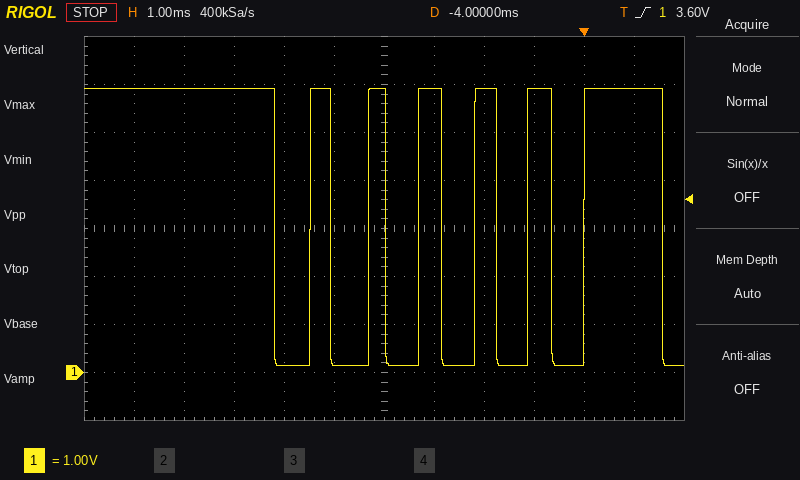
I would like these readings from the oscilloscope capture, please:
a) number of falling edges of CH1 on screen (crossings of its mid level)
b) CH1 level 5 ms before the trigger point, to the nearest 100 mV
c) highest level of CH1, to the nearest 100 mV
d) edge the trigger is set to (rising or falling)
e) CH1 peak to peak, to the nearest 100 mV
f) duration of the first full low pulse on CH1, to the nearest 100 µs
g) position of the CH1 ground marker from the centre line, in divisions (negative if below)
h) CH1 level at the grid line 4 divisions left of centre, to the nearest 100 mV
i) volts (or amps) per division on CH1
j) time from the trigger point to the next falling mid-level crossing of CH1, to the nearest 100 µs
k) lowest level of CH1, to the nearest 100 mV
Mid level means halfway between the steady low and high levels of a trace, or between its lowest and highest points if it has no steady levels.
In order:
7
200 mV
5.9 V
rising
5.8 V
700 µs
-3.0 div
5.9 V
1 V
1.6 ms
100 mV
